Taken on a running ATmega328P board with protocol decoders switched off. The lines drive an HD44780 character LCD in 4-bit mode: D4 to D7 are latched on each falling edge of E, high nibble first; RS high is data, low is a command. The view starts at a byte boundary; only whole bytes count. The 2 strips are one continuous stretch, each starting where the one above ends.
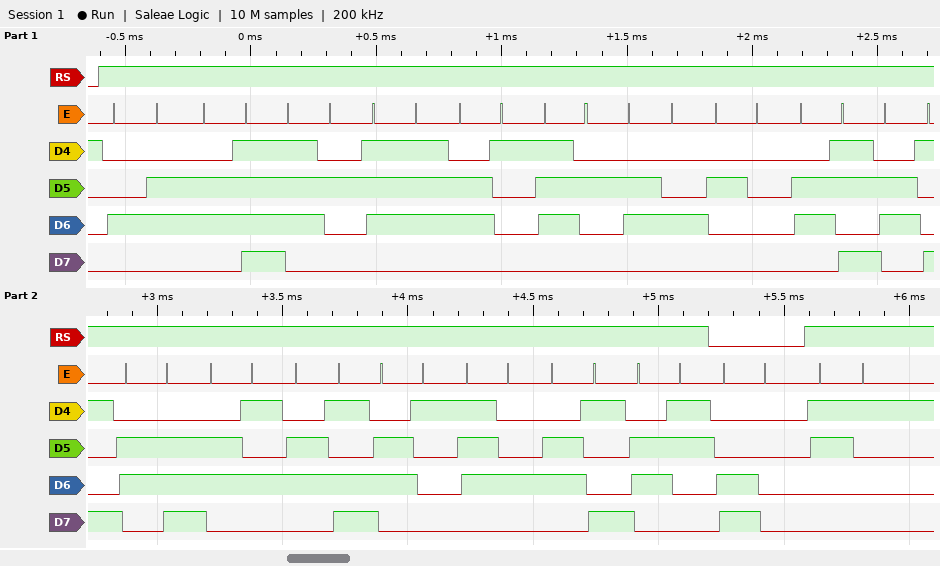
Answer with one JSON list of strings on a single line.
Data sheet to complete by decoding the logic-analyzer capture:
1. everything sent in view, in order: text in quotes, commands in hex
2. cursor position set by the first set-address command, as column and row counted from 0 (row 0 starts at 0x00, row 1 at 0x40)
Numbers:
["\"Forward kinematic\" 0xC0 \"1\"", "column 0, row 1"]
